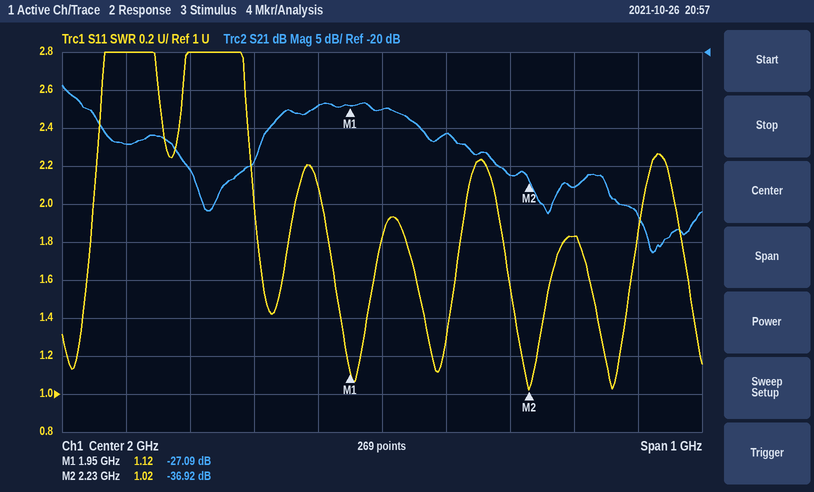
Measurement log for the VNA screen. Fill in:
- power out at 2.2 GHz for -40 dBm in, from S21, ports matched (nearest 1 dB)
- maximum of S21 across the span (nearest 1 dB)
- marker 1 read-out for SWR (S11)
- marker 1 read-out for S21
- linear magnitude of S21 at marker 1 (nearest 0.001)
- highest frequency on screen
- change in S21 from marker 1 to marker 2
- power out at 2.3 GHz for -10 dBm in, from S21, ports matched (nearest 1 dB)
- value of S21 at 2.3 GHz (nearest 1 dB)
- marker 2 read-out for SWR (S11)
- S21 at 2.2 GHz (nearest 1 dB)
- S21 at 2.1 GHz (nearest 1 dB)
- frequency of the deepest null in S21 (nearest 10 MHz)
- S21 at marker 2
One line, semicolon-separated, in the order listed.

-76 dBm; -24 dB; 1.12; -27.09 dB; 0.044; 2.5 GHz; -9.83 dB; -48 dBm; -38 dB; 1.02; -36 dB; -31 dB; 2.42 GHz; -36.92 dB
